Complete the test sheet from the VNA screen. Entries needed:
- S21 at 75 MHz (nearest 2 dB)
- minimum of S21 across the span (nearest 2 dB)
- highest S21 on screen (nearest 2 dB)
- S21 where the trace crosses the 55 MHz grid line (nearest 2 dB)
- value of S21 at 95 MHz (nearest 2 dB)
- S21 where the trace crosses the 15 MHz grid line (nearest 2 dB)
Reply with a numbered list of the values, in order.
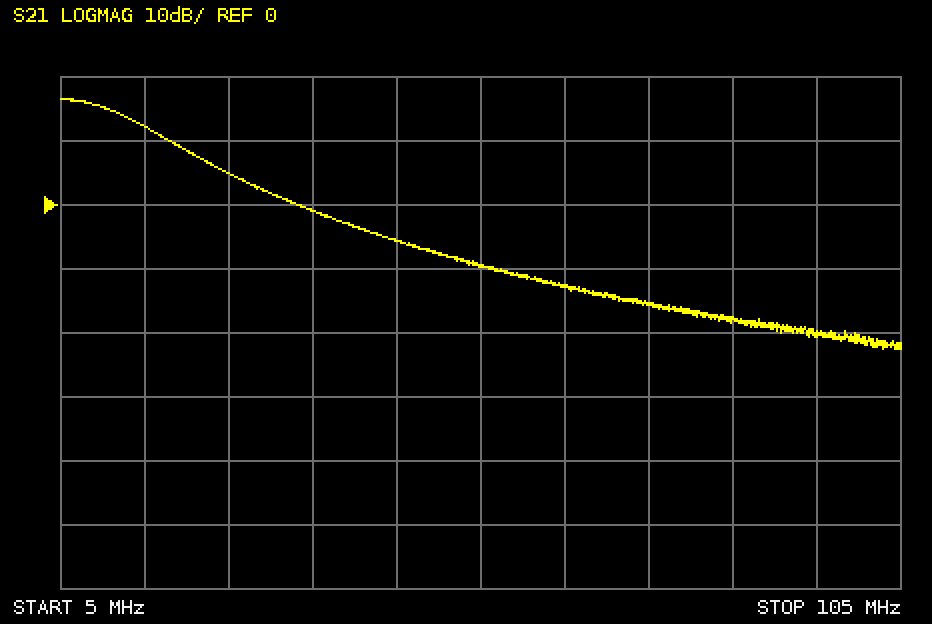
1. -16 dB
2. -22 dB
3. 16 dB
4. -10 dB
5. -20 dB
6. 12 dB
